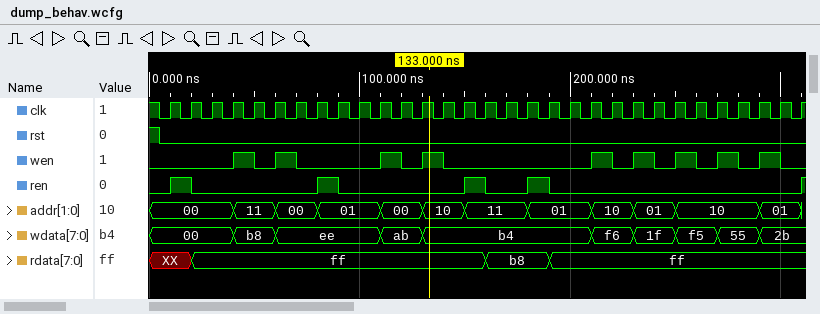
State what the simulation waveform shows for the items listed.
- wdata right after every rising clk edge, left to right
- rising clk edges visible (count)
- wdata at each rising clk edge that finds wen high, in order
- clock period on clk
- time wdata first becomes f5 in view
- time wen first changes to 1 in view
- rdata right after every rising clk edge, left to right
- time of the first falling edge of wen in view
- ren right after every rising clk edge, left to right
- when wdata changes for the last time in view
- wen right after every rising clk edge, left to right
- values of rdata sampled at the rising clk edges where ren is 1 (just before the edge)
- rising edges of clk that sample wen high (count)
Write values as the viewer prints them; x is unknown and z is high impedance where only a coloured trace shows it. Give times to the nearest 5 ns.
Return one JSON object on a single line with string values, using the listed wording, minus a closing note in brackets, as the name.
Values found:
{"wdata right after every rising clk edge, left to right": "00, 00, 00, b8, b8, ee, ee, ee, ee, ee, ab, ab, b4, b4, b4, b4, b4, b4, b4, b4, f6, f6, 1f, 1f, f5, f5, 55, 55, 2b, 2b, 2b", "rising clk edges visible": "31", "wdata at each rising clk edge that finds wen high, in order": "b8, ee, ab, b4, f6, 1f, f5, 55, 2b", "clock period on clk": "10 ns", "time wdata first becomes f5 in view": "250 ns", "time wen first changes to 1 in view": "40 ns", "rdata right after every rising clk edge, left to right": "XX, ff, ff, ff, ff, ff, ff, ff, ff, ff, ff, ff, ff, ff, ff, b8, b8, b8, ff, ff, ff, ff, ff, ff, ff, ff, ff, ff, ff, ff, ff", "time of the first falling edge of wen in view": "50 ns", "ren right after every rising clk edge, left to right": "1 0 0 0 0 0 0 1 0 0 0 0 0 0 1 0 0 1 0 0 0 0 0 0 0 0 0 0 0 0 1", "when wdata changes for the last time in view": "290 ns", "wen right after every rising clk edge, left to right": "0 0 0 1 0 1 0 0 0 0 1 0 1 0 0 0 0 0 0 0 1 0 1 0 1 0 1 0 1 0 0", "values of rdata sampled at the rising clk edges where ren is 1": "XX, ff, ff, b8", "rising edges of clk that sample wen high": "9"}
